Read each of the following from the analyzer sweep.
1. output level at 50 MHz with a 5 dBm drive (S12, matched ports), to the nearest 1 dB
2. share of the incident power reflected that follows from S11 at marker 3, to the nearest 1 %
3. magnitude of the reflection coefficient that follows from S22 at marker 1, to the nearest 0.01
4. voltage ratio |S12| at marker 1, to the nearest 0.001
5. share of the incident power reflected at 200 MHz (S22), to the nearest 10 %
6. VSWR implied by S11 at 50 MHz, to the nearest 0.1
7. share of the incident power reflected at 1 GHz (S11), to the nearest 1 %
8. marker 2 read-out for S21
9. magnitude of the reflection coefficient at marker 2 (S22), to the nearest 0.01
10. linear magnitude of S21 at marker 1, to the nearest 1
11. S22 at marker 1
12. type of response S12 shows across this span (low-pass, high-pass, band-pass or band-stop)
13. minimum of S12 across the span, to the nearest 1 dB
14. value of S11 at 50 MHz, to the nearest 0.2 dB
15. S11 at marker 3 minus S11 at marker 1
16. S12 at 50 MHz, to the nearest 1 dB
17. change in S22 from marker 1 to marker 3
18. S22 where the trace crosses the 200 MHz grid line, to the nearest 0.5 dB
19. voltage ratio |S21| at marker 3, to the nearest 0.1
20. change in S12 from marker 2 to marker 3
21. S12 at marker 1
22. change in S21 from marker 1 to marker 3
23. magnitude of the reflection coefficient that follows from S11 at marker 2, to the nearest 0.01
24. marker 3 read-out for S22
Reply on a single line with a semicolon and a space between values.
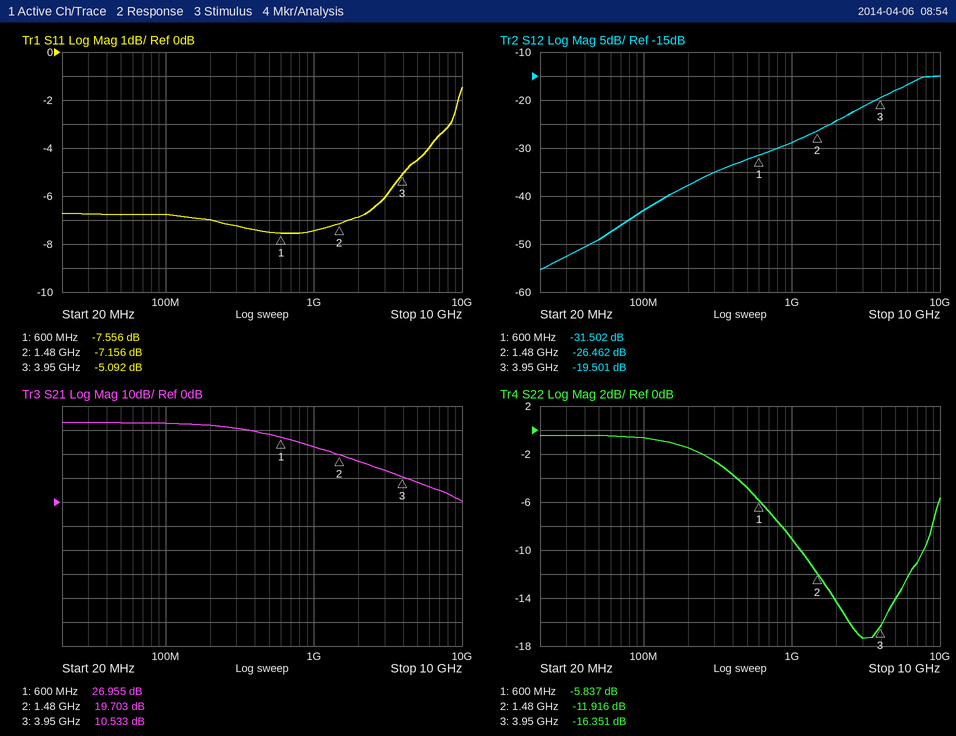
-44 dBm; 31 %; 0.51; 0.027; 70 %; 2.7; 18 %; 19.703 dB; 0.25; 22; -5.837 dB; high-pass; -55 dB; -6.8 dB; 2.464 dB; -49 dB; -10.514 dB; -1.5 dB; 3.4; 6.961 dB; -31.502 dB; -16.422 dB; 0.44; -16.351 dB
